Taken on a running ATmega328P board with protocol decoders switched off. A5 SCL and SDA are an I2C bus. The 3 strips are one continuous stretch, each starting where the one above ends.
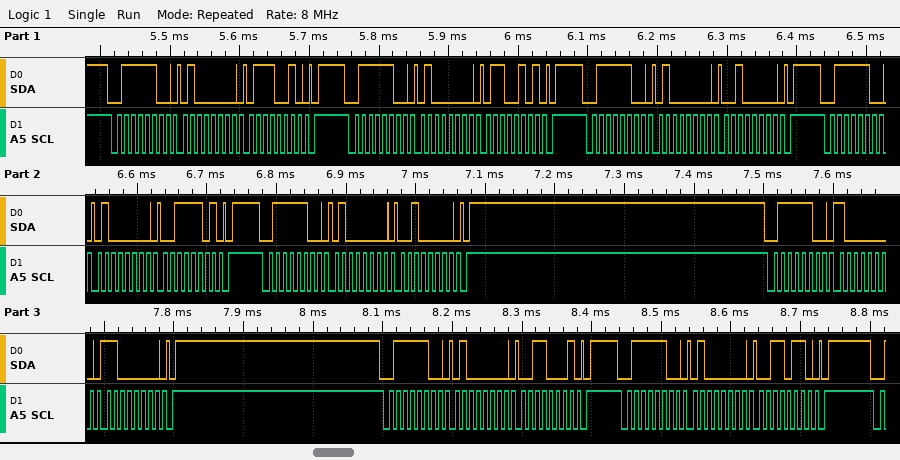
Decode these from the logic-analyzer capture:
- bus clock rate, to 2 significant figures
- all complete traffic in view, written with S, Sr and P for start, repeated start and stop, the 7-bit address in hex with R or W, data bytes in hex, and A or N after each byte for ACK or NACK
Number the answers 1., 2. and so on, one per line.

1. 100 kHz
2. S 3EW A 40 A 72 A P S 3EW A 40 A 65 A P S 3EW A 40 A 20 A P S 3EW A 40 A 3D A P S 3EW A 40 A 20 A P S 3EW A 80 A C0 A P S 3EW A 40 A 31 A P S 3EW A 40 A 36 A P
